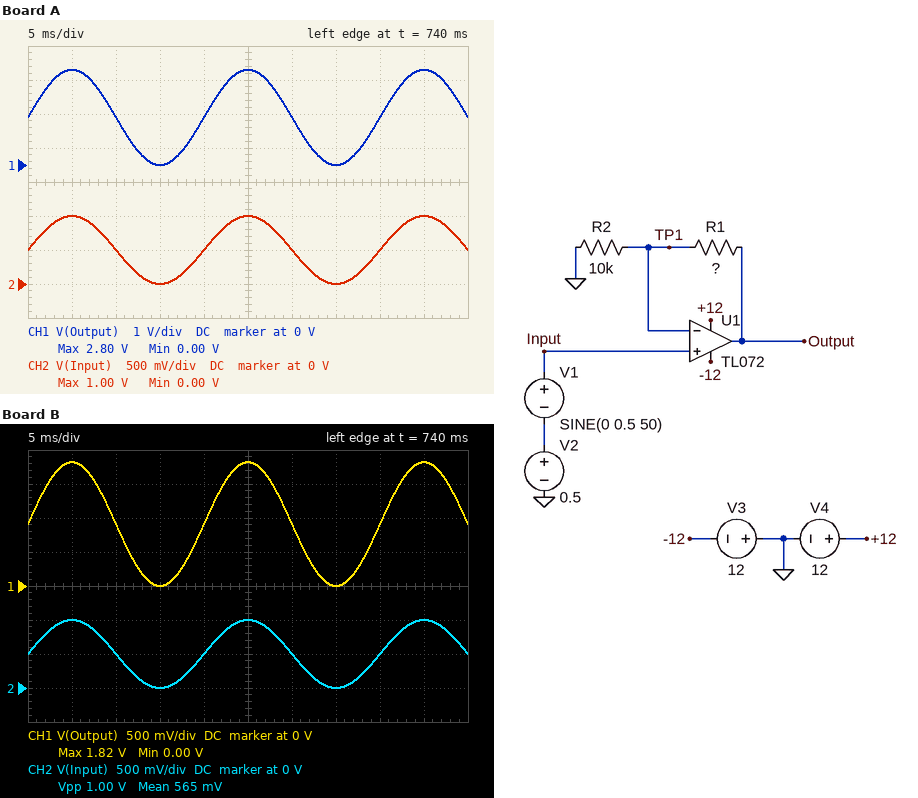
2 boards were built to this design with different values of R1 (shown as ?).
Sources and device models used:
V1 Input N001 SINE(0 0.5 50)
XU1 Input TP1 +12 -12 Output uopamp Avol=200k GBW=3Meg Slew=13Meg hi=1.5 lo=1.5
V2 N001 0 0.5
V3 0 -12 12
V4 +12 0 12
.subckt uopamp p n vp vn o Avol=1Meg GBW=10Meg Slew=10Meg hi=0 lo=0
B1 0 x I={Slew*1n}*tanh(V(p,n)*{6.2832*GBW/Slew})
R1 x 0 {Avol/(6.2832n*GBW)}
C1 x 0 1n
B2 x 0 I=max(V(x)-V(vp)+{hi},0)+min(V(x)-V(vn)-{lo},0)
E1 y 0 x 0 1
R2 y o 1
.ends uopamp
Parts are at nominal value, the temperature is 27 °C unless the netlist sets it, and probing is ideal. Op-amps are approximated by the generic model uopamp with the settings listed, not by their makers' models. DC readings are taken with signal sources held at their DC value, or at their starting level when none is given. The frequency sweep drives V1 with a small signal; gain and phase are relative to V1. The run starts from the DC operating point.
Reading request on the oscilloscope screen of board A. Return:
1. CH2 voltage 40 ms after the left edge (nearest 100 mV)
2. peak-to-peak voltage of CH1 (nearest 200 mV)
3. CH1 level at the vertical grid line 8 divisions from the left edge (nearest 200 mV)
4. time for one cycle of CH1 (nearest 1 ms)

500 mV
2.8 V
1.4 V
20 ms
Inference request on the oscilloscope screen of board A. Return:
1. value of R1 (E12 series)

18 kΩ
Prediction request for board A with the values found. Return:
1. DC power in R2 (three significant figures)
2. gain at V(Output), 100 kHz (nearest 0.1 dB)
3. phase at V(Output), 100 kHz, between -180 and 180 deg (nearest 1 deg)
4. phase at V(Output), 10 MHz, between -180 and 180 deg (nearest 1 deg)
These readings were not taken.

25.0 µW
8.9 dB
-5 deg
-84 deg
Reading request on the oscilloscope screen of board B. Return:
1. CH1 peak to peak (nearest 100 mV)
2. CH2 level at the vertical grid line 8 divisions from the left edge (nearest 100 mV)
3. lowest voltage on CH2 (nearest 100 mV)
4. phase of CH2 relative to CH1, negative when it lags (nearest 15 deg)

1.8 V
500 mV
0 V
0 deg
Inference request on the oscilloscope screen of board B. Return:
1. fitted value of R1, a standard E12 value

8.2 kΩ
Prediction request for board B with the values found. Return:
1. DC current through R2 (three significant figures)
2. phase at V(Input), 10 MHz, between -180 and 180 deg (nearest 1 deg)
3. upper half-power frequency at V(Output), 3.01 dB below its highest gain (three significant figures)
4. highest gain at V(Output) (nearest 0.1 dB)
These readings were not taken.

50.0 µA
0 deg
1.65 MHz
5.2 dB
